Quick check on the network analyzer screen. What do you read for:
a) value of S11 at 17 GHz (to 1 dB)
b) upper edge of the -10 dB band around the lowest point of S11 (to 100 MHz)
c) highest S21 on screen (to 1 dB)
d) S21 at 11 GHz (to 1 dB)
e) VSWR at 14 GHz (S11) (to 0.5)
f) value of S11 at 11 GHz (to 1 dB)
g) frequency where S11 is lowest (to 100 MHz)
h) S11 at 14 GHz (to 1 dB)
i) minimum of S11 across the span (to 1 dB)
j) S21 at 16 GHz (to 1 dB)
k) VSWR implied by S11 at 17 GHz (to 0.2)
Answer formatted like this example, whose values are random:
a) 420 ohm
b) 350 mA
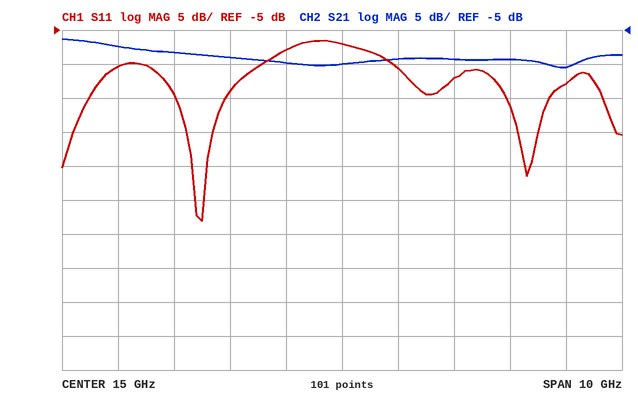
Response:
a) -12 dB
b) 13.6 GHz
c) -6 dB
d) -7 dB
e) 2.5
f) -10 dB
g) 12.5 GHz
h) -8 dB
i) -33 dB
j) -9 dB
k) 1.6
